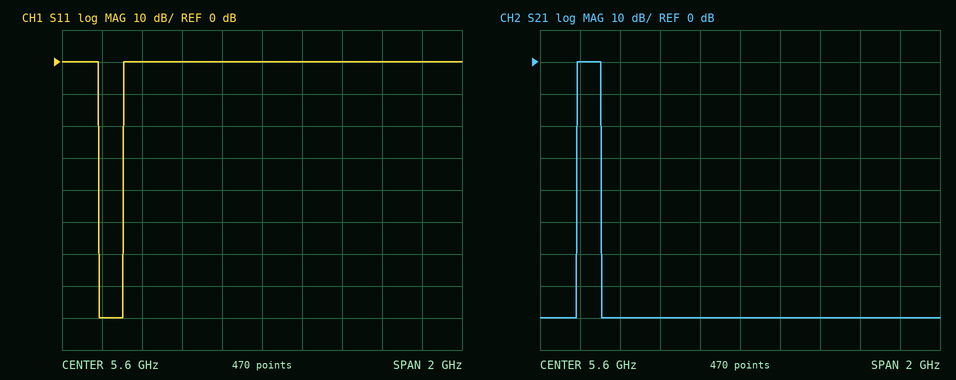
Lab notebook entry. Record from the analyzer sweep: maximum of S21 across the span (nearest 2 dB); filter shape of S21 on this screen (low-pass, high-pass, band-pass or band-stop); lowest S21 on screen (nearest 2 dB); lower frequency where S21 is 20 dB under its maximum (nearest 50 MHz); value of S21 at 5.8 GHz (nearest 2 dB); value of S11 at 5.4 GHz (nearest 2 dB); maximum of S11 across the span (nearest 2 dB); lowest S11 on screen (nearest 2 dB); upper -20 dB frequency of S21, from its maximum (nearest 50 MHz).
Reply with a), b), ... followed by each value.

a) 0 dB
b) band-pass
c) -80 dB
d) 4.80 GHz
e) -80 dB
f) 0 dB
g) 0 dB
h) -80 dB
i) 4.90 GHz
